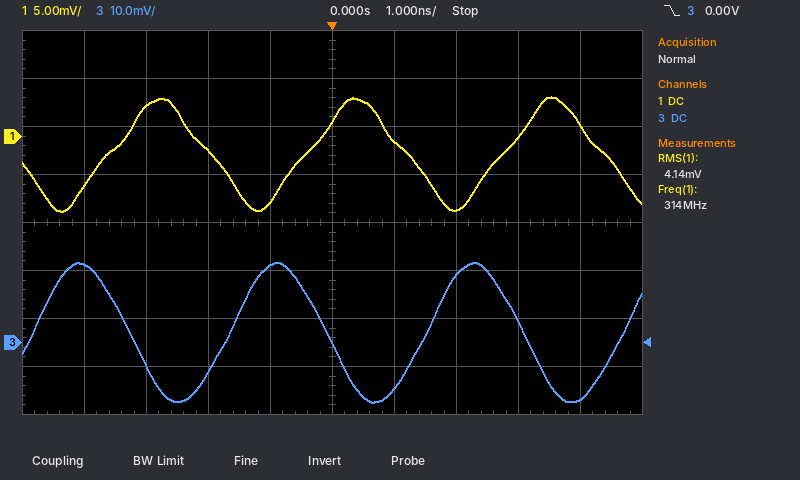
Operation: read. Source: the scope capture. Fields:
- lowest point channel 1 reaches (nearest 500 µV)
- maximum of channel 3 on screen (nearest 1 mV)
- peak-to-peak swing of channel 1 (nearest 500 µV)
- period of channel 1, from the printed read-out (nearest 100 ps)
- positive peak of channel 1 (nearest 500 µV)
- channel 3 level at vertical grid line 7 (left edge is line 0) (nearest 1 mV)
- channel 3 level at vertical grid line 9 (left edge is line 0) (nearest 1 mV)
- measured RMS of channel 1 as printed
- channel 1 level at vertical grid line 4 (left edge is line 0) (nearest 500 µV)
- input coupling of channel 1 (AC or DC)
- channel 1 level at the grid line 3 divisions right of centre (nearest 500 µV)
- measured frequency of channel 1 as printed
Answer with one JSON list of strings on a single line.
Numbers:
["-8.0 mV", "17 mV", "12.0 mV", "3.2 ns", "4.0 mV", "14 mV", "-12 mV", "4.14 mV", "-7.0 mV", "DC", "0.0 mV", "314 MHz"]
